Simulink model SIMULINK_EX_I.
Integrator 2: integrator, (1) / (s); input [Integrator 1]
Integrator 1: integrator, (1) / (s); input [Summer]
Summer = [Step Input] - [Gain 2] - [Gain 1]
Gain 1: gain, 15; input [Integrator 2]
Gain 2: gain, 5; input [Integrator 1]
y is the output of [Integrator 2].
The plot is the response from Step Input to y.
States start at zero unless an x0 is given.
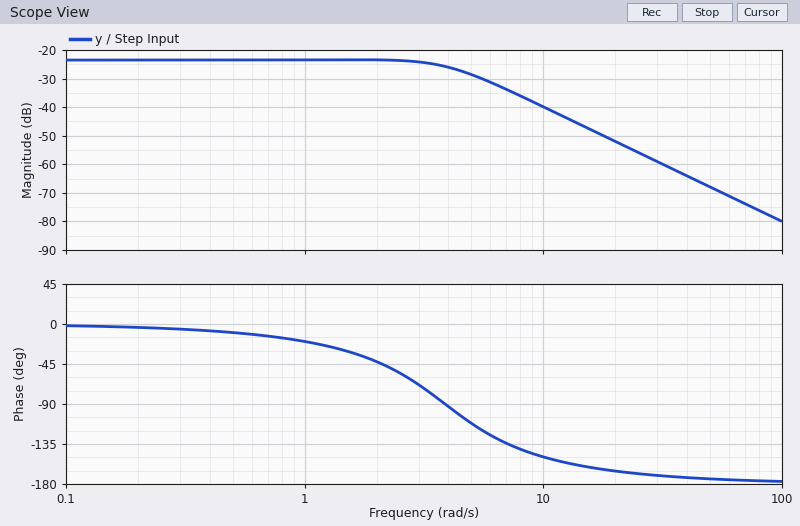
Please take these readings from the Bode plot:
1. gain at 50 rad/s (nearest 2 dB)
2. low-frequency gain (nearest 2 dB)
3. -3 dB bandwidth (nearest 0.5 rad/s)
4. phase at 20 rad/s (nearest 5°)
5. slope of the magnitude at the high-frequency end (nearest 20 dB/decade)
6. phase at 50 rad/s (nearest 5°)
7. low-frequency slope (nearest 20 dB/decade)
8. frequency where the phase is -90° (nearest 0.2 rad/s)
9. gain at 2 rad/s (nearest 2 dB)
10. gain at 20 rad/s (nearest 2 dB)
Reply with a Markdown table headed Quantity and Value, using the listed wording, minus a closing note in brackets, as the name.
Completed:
| Quantity | Value |
|---|---|
| gain at 50 rad/s | -68 dB |
| low-frequency gain | -24 dB |
| -3 dB bandwidth | 4.0 rad/s |
| phase at 20 rad/s | -165° |
| slope of the magnitude at the high-frequency end | -40 dB/decade |
| phase at 50 rad/s | -175° |
| low-frequency slope | 0 dB/decade |
| frequency where the phase is -90° | 3.8 rad/s |
| gain at 2 rad/s | -24 dB |
| gain at 20 rad/s | -52 dB |
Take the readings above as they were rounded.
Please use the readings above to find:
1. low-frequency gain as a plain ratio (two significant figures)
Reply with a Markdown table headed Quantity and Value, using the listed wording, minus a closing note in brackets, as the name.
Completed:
| Quantity | Value |
|---|---|
| low-frequency gain as a plain ratio | 0.063 |
